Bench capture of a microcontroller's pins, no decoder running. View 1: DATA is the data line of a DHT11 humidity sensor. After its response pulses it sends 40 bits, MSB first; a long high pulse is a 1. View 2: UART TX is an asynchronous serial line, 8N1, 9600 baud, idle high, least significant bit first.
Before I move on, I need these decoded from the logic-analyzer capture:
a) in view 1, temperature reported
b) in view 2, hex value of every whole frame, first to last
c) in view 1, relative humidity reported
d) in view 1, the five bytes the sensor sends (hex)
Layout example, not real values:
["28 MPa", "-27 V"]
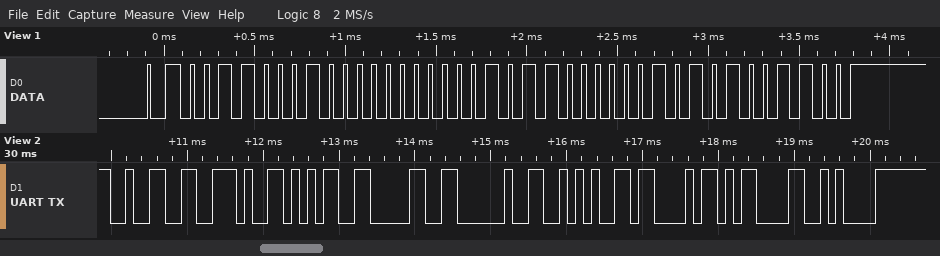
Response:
["22.5 °C", "0x32 0x2E 0x35 0x30 0x20 0x2A 0x43 0x0D 0x0A", "49 %", "31 00 16 05 4C"]
